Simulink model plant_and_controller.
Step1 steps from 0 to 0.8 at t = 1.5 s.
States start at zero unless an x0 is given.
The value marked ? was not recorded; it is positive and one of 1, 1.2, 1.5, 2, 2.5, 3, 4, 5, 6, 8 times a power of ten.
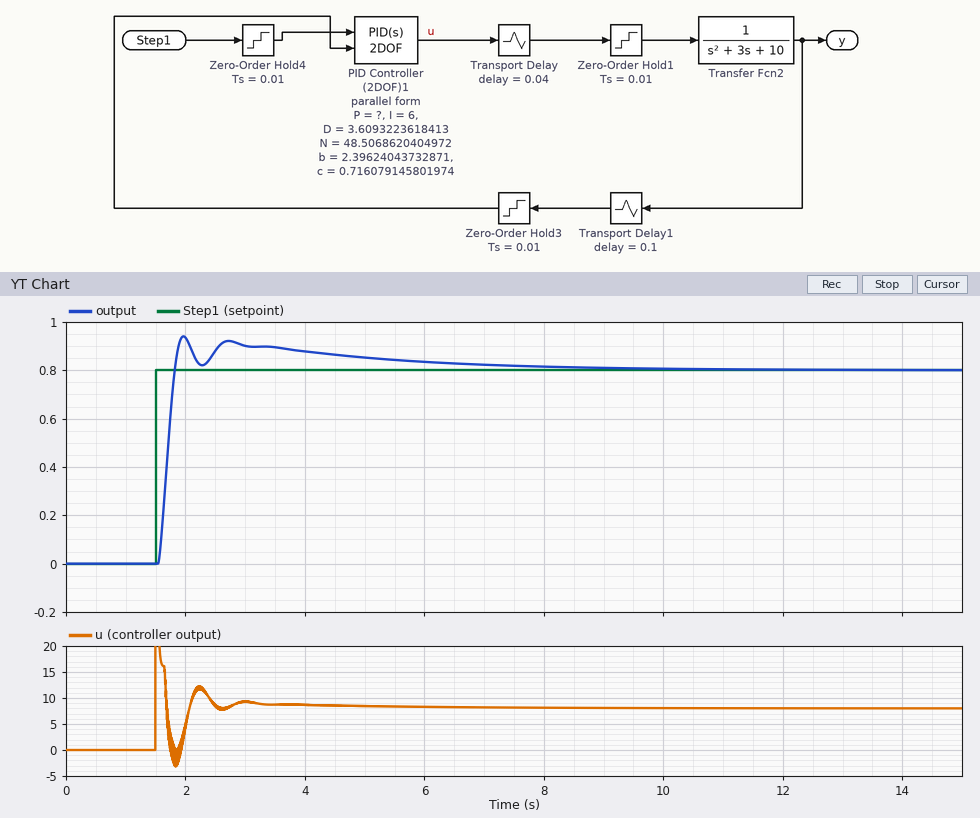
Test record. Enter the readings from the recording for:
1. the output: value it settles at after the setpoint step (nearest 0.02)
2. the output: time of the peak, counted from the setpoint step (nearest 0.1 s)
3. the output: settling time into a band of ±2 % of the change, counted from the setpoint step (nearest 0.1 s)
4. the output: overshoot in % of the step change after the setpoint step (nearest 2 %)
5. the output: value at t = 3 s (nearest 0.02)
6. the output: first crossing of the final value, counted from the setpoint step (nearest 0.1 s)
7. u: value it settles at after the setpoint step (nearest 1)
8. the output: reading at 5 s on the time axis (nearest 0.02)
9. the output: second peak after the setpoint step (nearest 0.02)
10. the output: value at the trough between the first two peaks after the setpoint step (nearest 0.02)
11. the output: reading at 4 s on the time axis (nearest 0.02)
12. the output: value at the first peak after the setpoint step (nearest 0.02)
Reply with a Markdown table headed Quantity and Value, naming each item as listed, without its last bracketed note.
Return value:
| Quantity | Value |
|---|---|
| the output: value it settles at after the setpoint step | 0.80 |
| the output: time of the peak, counted from the setpoint step | 0.5 s |
| the output: settling time into a band of ±2 % of the change, counted from the setpoint step | 6.4 s |
| the output: overshoot in % of the step change after the setpoint step | 18 % |
| the output: value at t = 3 s | 0.90 |
| the output: first crossing of the final value, counted from the setpoint step | 0.3 s |
| u: value it settles at after the setpoint step | 8 |
| the output: reading at 5 s on the time axis | 0.86 |
| the output: second peak after the setpoint step | 0.92 |
| the output: value at the trough between the first two peaks after the setpoint step | 0.82 |
| the output: reading at 4 s on the time axis | 0.88 |
| the output: value at the first peak after the setpoint step | 0.94 |
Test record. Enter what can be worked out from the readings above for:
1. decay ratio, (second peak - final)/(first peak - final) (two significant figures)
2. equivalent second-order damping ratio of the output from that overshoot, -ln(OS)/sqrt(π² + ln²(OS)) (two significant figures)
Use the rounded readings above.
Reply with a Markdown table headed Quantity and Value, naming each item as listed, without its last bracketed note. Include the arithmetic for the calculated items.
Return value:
| Quantity | Value |
|---|---|
| decay ratio, (second peak - final)/(first peak - final) | (0.92 - 0.8) / (0.94 - 0.8) = 0.86 |
| equivalent second-order damping ratio of the output from that overshoot, -ln(OS)/sqrt(π² + ln²(OS)) | ln(0.18) = -1.715; 1.715 / sqrt(9.870 + 2.941) = 0.48 |
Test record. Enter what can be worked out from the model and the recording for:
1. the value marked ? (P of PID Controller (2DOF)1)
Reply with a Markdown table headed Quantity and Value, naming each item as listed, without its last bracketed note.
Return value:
| Quantity | Value |
|---|---|
| the value marked ? (P of PID Controller (2DOF)1) | 8 |
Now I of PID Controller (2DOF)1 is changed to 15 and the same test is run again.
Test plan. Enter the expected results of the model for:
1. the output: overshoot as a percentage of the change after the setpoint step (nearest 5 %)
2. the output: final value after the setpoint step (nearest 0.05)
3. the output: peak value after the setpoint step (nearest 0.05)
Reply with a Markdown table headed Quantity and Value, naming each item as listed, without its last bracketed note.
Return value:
| Quantity | Value |
|---|---|
| the output: overshoot as a percentage of the change after the setpoint step | 25 % |
| the output: final value after the setpoint step | 0.80 |
| the output: peak value after the setpoint step | 1.00 |
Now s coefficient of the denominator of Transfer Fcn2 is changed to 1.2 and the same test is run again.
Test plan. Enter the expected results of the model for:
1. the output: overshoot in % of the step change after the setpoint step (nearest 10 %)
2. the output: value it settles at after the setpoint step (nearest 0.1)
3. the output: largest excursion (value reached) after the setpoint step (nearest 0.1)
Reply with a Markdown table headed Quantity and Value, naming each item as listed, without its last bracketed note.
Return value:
| Quantity | Value |
|---|---|
| the output: overshoot in % of the step change after the setpoint step | 50 % |
| the output: value it settles at after the setpoint step | 0.8 |
| the output: largest excursion (value reached) after the setpoint step | 1.2 |
